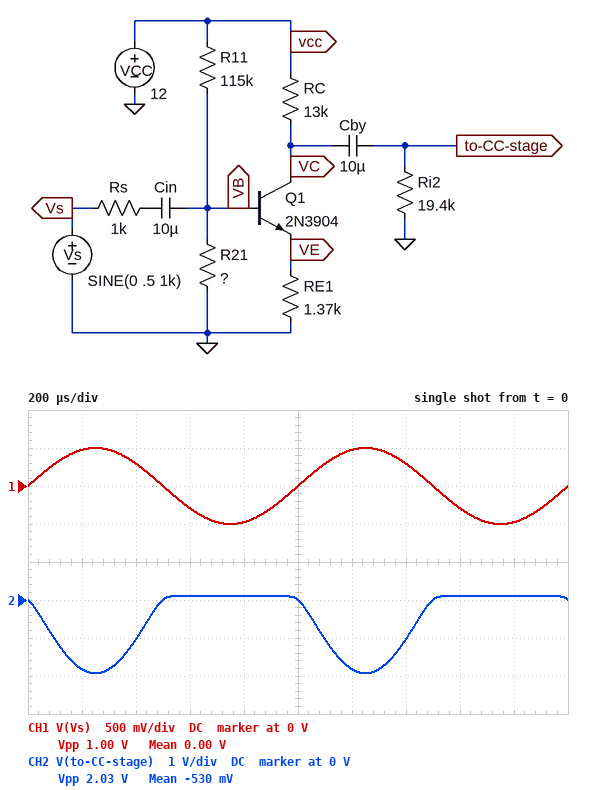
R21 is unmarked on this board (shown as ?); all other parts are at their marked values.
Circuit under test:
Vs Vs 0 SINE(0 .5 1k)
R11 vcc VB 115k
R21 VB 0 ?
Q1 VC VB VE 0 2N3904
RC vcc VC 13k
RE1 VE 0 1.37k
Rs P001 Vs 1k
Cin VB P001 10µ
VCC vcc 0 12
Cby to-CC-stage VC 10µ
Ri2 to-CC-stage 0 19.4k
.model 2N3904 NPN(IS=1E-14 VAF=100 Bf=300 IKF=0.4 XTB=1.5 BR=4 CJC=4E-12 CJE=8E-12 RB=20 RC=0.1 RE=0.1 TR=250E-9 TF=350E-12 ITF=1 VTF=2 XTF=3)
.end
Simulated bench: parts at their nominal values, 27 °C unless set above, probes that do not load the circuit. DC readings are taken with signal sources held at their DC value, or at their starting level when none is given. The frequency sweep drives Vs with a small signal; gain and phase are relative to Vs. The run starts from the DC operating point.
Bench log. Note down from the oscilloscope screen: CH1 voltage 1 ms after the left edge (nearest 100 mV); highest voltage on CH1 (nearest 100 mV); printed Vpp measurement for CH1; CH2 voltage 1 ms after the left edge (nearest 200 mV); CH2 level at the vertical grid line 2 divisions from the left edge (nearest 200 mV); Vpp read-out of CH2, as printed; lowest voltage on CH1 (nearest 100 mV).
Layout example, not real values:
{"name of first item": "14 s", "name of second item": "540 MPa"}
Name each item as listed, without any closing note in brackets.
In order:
{"CH1 voltage 1 ms after the left edge": "0 V", "highest voltage on CH1": "500 mV", "printed Vpp measurement for CH1": "1.00 V", "CH2 voltage 1 ms after the left edge": "0 V", "CH2 level at the vertical grid line 2 divisions from the left edge": "-1.0 V", "Vpp read-out of CH2, as printed": "2.03 V", "lowest voltage on CH1": "-500 mV"}
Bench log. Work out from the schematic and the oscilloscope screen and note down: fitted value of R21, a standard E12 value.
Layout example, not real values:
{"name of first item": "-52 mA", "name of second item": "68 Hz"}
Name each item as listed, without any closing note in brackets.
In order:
{"fitted value of R21, a standard E12 value": "5.6 kΩ"}
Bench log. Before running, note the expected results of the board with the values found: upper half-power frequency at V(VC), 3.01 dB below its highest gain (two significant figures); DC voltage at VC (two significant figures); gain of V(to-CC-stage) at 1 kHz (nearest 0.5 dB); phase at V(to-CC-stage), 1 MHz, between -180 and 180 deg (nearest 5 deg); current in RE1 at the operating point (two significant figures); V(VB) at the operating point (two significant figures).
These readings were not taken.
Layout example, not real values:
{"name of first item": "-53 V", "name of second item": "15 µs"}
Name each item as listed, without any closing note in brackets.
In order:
{"upper half-power frequency at V(VC), 3.01 dB below its highest gain": "7.4 MHz", "DC voltage at VC": "12 V", "gain of V(to-CC-stage) at 1 kHz": "5.5 dB", "phase at V(to-CC-stage), 1 MHz, between -180 and 180 deg": "165 deg", "current in RE1 at the operating point": "13 µA", "V(VB) at the operating point": "560 mV"}
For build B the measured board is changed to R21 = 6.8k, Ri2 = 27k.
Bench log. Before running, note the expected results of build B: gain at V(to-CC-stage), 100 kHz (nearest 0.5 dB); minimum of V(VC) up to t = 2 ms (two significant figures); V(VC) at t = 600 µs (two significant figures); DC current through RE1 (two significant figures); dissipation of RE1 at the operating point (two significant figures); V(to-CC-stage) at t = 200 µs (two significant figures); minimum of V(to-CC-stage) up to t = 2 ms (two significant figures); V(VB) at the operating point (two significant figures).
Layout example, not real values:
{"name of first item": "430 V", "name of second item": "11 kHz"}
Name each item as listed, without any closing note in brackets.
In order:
{"gain at V(to-CC-stage), 100 kHz": "12.5 dB", "minimum of V(VC) up to t = 2 ms": "8.7 V", "V(VC) at t = 600 µs": "12 V", "DC current through RE1": "64 µA", "dissipation of RE1 at the operating point": "5.6 µW", "V(to-CC-stage) at t = 200 µs": "-2.3 V", "minimum of V(to-CC-stage) up to t = 2 ms": "-2.5 V", "V(VB) at the operating point": "670 mV"}
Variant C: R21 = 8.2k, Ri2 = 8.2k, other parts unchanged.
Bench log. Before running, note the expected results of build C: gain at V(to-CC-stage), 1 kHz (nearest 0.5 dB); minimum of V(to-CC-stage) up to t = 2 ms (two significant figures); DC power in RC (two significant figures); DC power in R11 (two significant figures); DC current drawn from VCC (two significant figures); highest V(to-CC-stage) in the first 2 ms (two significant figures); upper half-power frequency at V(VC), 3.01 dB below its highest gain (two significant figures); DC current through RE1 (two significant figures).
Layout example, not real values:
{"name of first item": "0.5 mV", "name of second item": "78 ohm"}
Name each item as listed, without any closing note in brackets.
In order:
{"gain at V(to-CC-stage), 1 kHz": "9.0 dB", "minimum of V(to-CC-stage) up to t = 2 ms": "-1.5 V", "DC power in RC": "260 µW", "DC power in R11": "1.1 mW", "DC current drawn from VCC": "240 µA", "highest V(to-CC-stage) in the first 2 ms": "710 mV", "upper half-power frequency at V(VC), 3.01 dB below its highest gain": "10 MHz", "DC current through RE1": "140 µA"}
